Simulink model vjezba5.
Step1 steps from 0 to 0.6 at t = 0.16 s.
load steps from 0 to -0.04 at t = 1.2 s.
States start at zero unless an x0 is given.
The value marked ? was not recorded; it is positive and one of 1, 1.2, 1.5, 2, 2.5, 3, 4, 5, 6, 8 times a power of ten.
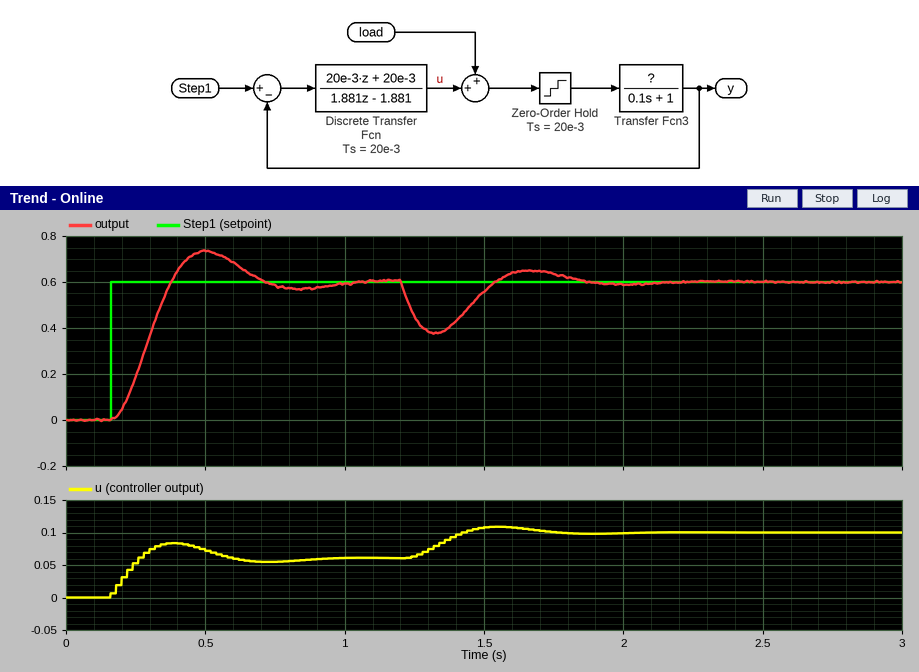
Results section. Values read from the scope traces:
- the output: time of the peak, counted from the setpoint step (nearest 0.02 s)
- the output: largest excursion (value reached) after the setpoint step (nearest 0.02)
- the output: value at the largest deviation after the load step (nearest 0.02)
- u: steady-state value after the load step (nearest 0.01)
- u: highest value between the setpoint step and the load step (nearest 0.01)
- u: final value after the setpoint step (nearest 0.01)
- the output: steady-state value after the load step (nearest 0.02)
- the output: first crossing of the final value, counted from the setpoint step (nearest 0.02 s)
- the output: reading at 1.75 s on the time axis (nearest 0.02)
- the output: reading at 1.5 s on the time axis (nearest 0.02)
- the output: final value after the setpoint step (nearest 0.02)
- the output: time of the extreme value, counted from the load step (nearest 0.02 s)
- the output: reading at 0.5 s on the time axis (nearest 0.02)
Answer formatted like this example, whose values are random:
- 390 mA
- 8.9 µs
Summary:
- 0.34 s
- 0.74
- 0.38
- 0.10
- 0.08
- 0.06
- 0.60
- 0.22 s
- 0.64
- 0.56
- 0.60
- 0.12 s
- 0.74
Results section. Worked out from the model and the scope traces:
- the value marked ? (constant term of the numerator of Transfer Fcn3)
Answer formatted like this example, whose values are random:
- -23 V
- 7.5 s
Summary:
- 10
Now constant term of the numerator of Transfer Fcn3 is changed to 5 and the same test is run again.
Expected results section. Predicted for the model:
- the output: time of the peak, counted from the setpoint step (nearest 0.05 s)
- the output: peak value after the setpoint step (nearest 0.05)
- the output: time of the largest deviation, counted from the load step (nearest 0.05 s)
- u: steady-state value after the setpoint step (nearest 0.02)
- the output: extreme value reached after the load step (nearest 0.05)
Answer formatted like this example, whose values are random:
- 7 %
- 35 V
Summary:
- 0.55 s
- 0.65
- 0.15 s
- 0.12
- 0.45
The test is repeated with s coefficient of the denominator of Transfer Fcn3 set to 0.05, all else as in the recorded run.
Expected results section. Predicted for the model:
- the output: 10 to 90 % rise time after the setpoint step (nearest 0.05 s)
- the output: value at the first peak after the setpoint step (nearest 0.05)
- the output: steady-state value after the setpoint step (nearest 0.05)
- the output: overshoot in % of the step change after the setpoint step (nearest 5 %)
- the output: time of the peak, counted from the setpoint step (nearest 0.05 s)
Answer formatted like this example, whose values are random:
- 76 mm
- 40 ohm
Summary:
- 0.15 s
- 0.65
- 0.60
- 10 %
- 0.30 s
